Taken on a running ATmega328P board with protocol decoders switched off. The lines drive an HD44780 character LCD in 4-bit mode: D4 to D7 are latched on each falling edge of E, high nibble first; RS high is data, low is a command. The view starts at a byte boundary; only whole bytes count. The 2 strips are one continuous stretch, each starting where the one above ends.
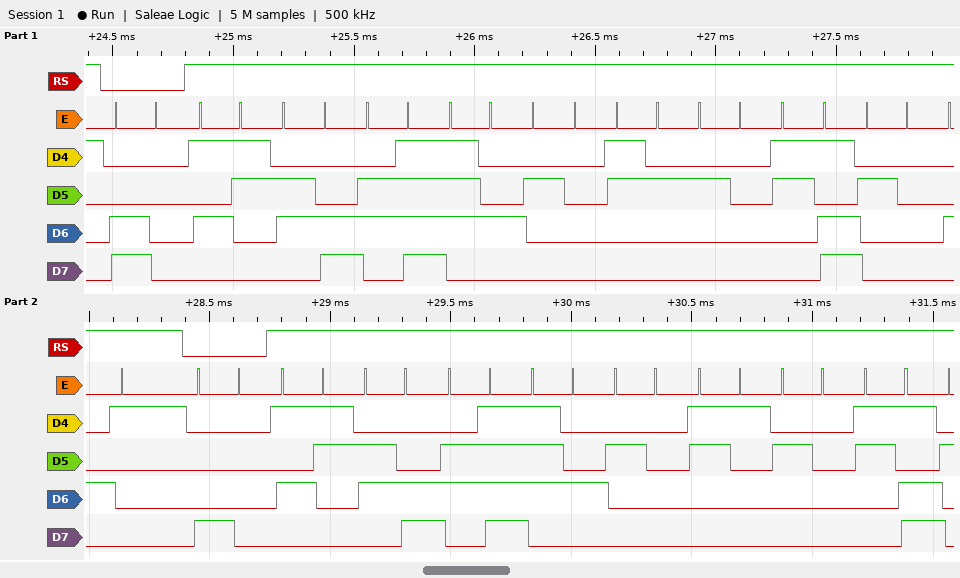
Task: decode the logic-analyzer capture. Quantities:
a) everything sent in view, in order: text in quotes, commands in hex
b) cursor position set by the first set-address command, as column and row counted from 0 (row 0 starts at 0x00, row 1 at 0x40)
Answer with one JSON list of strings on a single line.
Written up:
["0xC0 \"Slot 2 = A\" 0x80 \"Slot 1 =\"", "column 0, row 1"]
